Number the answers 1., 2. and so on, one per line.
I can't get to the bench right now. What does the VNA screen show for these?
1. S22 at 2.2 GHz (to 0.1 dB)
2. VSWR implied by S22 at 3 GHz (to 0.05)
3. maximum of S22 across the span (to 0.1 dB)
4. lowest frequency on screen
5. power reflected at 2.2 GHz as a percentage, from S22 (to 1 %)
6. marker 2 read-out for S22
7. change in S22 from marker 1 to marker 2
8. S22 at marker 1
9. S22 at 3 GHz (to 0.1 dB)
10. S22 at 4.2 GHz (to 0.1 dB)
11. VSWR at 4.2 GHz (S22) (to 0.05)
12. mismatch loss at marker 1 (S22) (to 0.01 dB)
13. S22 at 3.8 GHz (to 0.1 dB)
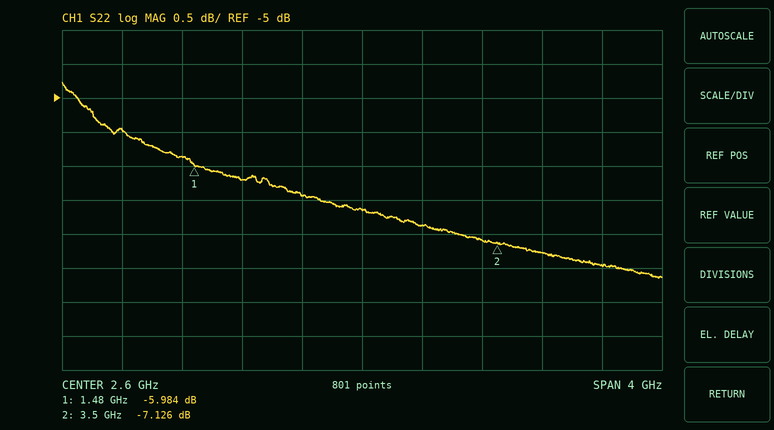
1. -6.4 dB
2. 2.65
3. -4.8 dB
4. 600 MHz
5. 23 %
6. -7.126 dB
7. -1.142 dB
8. -5.984 dB
9. -6.9 dB
10. -7.5 dB
11. 2.45
12. 1.26 dB
13. -7.3 dB
